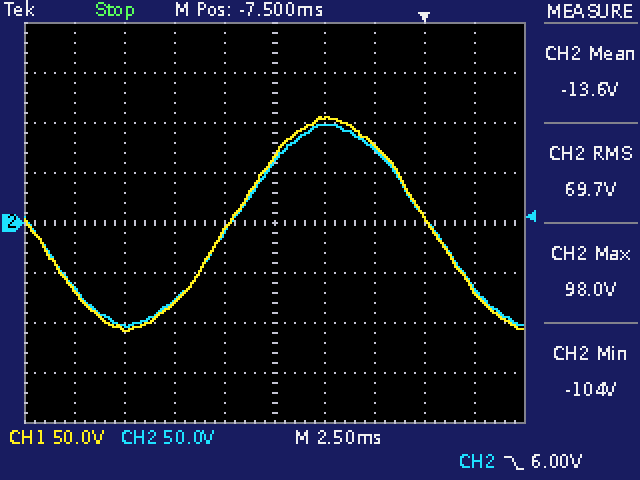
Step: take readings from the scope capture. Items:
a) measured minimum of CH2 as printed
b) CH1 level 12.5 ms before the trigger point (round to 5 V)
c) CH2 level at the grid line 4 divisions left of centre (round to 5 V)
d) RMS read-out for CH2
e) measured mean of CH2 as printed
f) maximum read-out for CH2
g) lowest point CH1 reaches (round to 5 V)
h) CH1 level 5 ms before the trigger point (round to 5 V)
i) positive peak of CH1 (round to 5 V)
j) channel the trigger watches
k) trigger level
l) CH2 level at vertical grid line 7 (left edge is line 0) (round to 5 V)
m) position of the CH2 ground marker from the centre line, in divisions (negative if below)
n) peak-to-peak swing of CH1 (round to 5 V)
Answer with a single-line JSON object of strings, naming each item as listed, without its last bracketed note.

{"measured minimum of CH2 as printed": "-104 V", "CH1 level 12.5 ms before the trigger point": "-80 V", "CH2 level at the grid line 4 divisions left of centre": "-65 V", "RMS read-out for CH2": "69.7 V", "measured mean of CH2 as printed": "-13.6 V", "maximum read-out for CH2": "98.0 V", "lowest point CH1 reaches": "-110 V", "CH1 level 5 ms before the trigger point": "105 V", "positive peak of CH1": "105 V", "channel the trigger watches": "CH2", "trigger level": "6.00 V", "CH2 level at vertical grid line 7 (left edge is line 0)": "75 V", "position of the CH2 ground marker from the centre line, in divisions": "0.0 div", "peak-to-peak swing of CH1": "215 V"}
